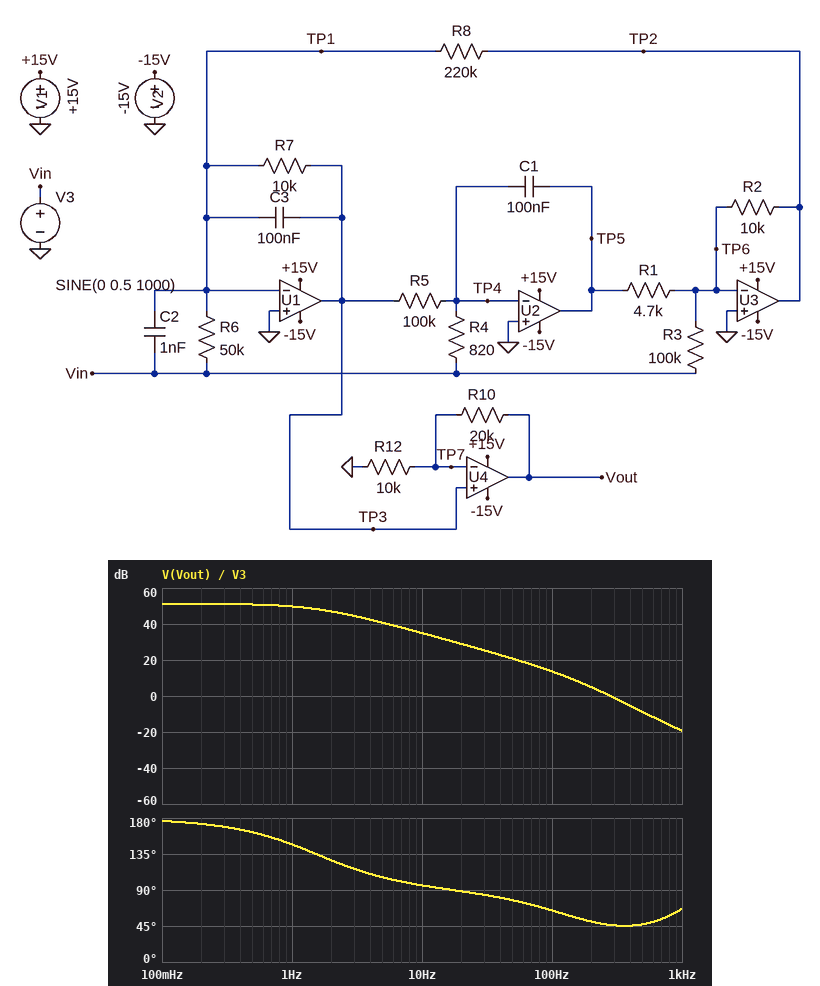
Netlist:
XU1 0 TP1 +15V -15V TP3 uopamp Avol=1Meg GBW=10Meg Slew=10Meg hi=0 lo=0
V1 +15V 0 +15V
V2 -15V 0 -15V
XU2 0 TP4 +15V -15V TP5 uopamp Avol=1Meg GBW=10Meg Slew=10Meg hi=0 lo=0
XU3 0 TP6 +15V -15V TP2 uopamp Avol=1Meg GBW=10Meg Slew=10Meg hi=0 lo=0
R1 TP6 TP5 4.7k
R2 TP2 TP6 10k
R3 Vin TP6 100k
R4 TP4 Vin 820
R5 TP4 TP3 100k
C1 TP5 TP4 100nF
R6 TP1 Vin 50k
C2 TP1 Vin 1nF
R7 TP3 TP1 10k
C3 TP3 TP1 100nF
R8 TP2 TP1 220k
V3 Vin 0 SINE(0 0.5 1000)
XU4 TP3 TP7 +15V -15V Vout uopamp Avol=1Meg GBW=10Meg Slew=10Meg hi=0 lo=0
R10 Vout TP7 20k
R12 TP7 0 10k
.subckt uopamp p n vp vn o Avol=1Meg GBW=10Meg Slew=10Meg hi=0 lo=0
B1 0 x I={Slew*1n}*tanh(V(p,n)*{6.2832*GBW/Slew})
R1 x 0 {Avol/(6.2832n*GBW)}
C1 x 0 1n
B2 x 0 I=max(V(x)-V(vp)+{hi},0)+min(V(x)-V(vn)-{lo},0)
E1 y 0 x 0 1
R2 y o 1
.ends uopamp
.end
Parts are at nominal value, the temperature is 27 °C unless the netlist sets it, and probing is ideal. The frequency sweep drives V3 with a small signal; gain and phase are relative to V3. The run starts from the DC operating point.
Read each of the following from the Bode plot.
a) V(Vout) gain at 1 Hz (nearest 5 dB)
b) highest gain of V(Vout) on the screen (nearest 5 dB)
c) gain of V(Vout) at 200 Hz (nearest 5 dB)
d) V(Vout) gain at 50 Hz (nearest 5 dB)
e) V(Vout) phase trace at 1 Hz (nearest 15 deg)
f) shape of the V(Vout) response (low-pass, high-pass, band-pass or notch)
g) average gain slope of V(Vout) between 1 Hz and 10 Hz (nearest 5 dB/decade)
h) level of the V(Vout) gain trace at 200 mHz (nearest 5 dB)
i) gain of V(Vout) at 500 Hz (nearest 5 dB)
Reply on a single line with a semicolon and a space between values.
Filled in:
50 dB; 50 dB; 5 dB; 20 dB; 150 deg; low-pass; -15 dB/decade; 50 dB; -10 dB
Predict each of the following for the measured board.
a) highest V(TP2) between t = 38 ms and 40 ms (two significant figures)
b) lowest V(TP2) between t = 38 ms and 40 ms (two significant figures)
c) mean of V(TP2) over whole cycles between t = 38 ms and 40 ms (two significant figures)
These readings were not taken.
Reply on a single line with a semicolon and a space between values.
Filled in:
3.5 V; -660 mV; 1.4 V
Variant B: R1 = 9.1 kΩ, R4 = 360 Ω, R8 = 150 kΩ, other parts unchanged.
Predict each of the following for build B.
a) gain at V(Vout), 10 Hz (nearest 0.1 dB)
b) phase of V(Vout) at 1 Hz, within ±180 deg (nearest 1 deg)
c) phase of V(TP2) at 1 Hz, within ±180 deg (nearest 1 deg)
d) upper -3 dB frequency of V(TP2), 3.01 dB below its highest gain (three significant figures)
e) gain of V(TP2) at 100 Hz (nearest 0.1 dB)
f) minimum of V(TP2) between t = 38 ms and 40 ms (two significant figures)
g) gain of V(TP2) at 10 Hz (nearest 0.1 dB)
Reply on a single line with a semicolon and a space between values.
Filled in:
39.7 dB; 139 deg; -40 deg; 1.18 Hz; 33.8 dB; -610 mV; 53.7 dB
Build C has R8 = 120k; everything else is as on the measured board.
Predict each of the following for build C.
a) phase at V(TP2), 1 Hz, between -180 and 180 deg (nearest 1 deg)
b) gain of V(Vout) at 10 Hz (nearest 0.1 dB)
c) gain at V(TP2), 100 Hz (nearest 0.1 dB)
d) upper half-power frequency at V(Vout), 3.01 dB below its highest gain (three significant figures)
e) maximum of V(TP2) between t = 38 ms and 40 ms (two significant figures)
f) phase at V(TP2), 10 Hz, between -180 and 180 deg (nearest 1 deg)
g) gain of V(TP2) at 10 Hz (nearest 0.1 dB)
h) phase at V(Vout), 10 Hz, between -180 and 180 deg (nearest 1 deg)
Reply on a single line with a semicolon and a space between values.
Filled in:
-19 deg; 40.1 dB; 32.4 dB; 2.87 Hz; 3.1 V; -74 deg; 52.1 dB; 103 deg
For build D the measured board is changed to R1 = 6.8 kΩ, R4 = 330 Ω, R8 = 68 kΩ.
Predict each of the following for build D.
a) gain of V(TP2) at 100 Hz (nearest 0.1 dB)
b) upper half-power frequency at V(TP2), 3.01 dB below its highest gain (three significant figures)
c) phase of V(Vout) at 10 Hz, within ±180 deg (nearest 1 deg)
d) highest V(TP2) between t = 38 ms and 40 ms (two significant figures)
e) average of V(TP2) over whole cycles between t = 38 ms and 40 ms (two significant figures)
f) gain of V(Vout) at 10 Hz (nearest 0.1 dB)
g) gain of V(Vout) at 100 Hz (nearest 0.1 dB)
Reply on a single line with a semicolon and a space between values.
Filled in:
37.1 dB; 3.52 Hz; 106 deg; 5.1 V; 1.5 V; 49.6 dB; 28.6 dB
